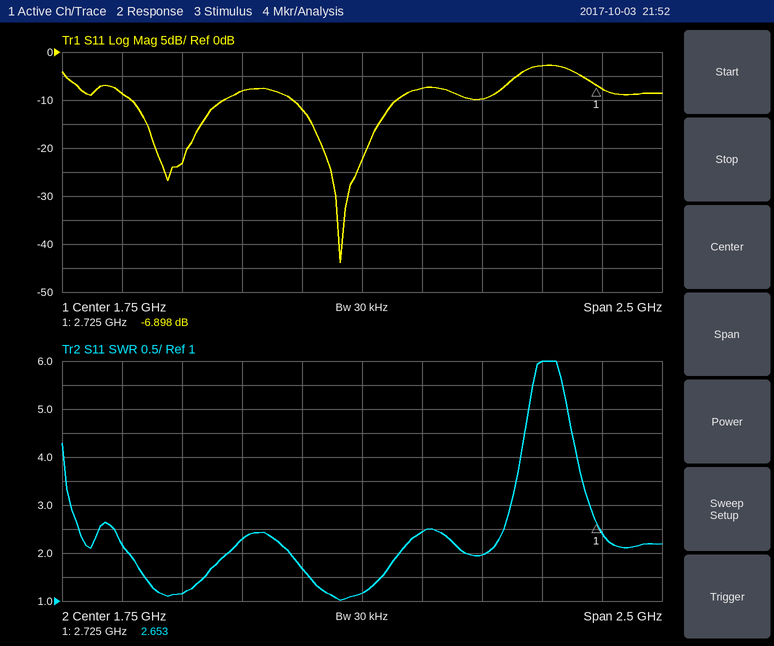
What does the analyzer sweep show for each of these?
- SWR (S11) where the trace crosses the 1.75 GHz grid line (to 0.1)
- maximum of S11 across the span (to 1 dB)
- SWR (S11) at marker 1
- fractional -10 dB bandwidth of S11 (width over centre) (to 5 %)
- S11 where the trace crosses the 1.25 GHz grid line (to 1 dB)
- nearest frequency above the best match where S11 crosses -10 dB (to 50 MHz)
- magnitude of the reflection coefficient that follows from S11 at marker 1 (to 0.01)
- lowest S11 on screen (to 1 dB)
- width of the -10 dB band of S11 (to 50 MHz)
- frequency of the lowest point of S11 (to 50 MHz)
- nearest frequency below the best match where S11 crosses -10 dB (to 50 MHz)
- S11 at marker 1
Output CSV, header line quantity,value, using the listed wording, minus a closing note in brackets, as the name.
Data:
quantity,value
SWR (S11) where the trace crosses the 1.75 GHz grid line,1.2
maximum of S11 across the span,-3 dB
SWR (S11) at marker 1,2.653
fractional -10 dB bandwidth of S11 (width over centre),25 %
S11 where the trace crosses the 1.25 GHz grid line,-8 dB
nearest frequency above the best match where S11 crosses -10 dB,1.90 GHz
magnitude of the reflection coefficient that follows from S11 at marker 1,0.45
lowest S11 on screen,-44 dB
width of the -10 dB band of S11,450 MHz
frequency of the lowest point of S11,1.65 GHz
nearest frequency below the best match where S11 crosses -10 dB,1.45 GHz
S11 at marker 1,-6.898 dB
